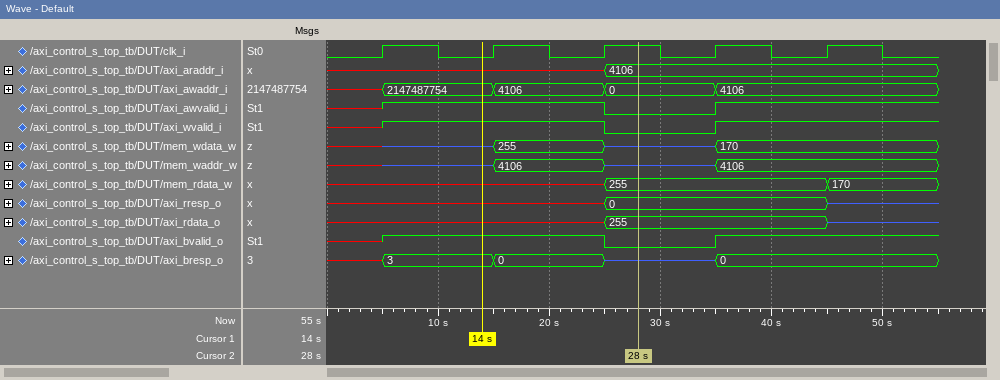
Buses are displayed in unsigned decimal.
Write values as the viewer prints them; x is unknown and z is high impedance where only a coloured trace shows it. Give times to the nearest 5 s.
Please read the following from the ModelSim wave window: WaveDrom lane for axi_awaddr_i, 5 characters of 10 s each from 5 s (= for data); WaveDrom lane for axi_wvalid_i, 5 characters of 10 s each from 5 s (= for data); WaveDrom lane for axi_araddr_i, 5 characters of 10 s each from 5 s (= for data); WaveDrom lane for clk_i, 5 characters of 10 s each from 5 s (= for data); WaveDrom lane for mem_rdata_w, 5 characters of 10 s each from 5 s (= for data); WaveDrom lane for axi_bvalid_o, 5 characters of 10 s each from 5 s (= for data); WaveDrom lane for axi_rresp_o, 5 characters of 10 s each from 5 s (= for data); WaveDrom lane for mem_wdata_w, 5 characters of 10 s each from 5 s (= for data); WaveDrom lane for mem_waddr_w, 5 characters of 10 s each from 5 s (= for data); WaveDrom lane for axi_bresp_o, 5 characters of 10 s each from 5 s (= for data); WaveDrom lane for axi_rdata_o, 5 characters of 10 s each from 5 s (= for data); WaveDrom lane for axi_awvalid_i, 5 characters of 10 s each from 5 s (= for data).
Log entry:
{name: 'axi_awaddr_i', wave: '====.', data: '2147487754 4106 0 4106'}
{name: 'axi_wvalid_i', wave: '1.01.'}
{name: 'axi_araddr_i', wave: 'x.=..', data: '4106'}
{name: 'clk_i', wave: 'p....'}
{name: 'mem_rdata_w', wave: 'x.=.=', data: '255 170'}
{name: 'axi_bvalid_o', wave: '1.01.'}
{name: 'axi_rresp_o', wave: 'x.=.z', data: '0'}
{name: 'mem_wdata_w', wave: 'z=z=.', data: '255 170'}
{name: 'mem_waddr_w', wave: 'z=z=.', data: '4106 4106'}
{name: 'axi_bresp_o', wave: '==z=.', data: '3 0 0'}
{name: 'axi_rdata_o', wave: 'x.=.z', data: '255'}
{name: 'axi_awvalid_i', wave: '1.01.'}
